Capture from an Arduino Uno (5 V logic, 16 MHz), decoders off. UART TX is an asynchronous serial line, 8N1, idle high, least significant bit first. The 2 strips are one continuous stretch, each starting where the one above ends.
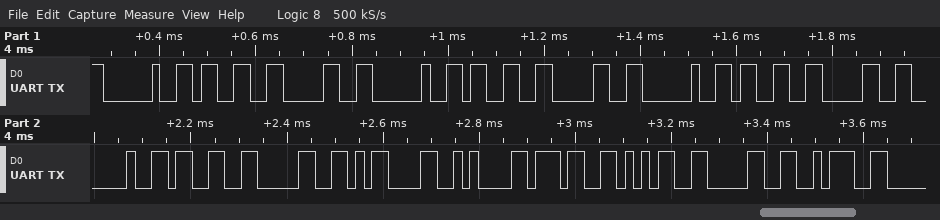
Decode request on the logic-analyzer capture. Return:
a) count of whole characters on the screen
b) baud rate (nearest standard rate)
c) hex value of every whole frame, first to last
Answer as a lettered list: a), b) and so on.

a) 18
b) 57600 baud
c) 20 33 30 20 33 30 20 33 30 20 33 30 0D 0A 37 35 30 3A
